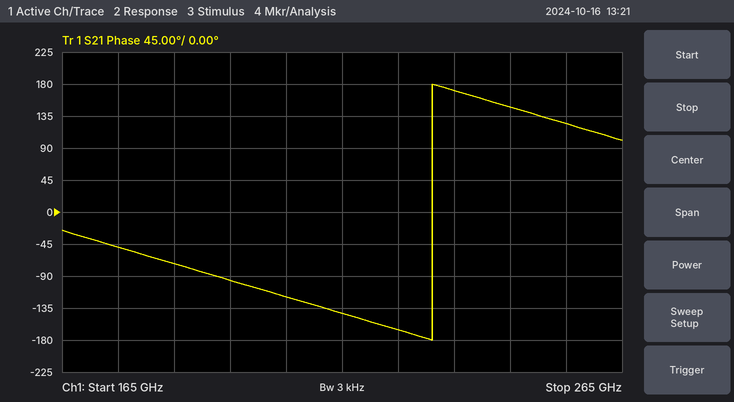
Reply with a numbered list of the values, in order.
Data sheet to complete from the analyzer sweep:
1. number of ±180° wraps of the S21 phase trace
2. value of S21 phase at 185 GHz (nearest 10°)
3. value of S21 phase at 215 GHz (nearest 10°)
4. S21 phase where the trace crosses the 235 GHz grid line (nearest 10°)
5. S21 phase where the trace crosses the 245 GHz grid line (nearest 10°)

1. 1
2. -70°
3. -140°
4. 170°
5. 150°
